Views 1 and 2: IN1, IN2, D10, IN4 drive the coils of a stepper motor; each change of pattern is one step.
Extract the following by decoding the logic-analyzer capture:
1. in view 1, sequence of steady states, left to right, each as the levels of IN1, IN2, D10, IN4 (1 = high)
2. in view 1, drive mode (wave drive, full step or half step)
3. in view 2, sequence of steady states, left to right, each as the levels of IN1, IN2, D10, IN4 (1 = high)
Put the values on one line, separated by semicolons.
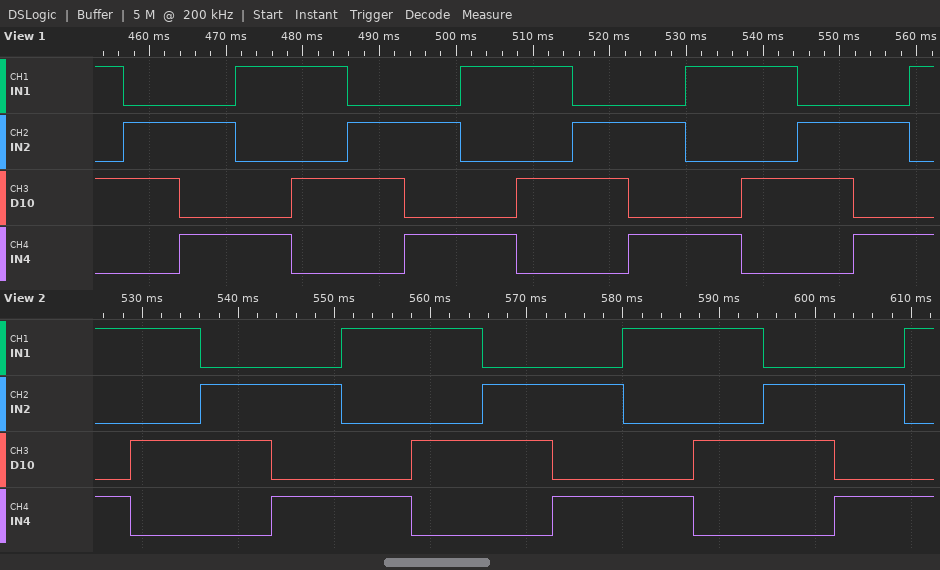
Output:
1010 0110 0101 1001 1010 0110 0101 1001 1010 0110 0101 1001 1010 0110 0101 1001; full step; 1001 1010 0110 0101 1001 1010 0110 0101 1001 1010 0110 0101 1001
